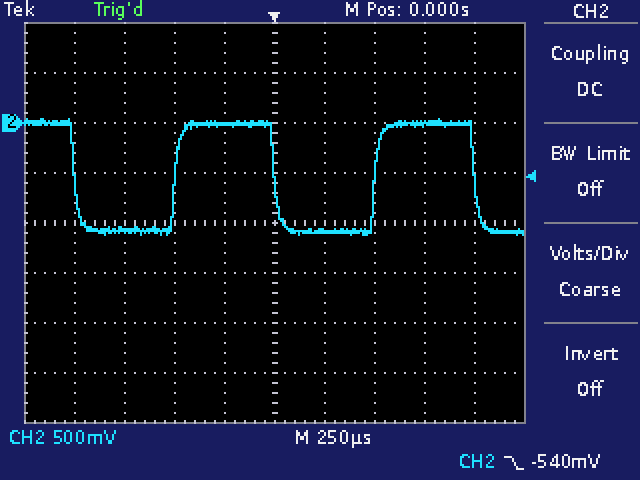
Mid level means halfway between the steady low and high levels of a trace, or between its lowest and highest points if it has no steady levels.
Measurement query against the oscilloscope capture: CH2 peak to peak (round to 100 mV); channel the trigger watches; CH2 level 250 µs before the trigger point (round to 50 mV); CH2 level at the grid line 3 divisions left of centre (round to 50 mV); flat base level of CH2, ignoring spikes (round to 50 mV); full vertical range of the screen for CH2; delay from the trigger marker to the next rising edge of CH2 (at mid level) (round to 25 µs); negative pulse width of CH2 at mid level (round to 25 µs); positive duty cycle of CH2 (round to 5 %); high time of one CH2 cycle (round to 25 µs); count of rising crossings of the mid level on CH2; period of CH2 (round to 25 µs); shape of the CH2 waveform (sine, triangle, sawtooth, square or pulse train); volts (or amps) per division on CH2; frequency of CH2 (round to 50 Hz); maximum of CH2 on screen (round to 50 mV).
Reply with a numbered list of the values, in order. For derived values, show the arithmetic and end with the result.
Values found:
1. 1.20 V
2. CH2
3. 0 mV
4. -1.05 V
5. -1.10 V
6. 4 V
7. 500 µs
8. 500 µs
9. 500 µs / 1.000 ms ≈ 50 %
10. 500 µs
11. 2
12. 1.000 ms
13. square
14. 500 mV
15. 1 / 1.000 ms ≈ 1.00 kHz
16. 50 mV
